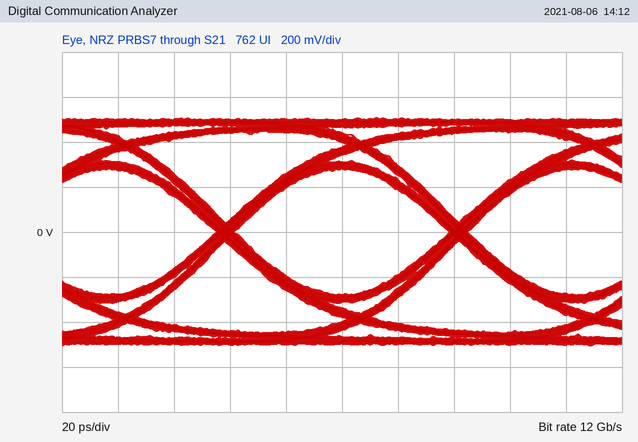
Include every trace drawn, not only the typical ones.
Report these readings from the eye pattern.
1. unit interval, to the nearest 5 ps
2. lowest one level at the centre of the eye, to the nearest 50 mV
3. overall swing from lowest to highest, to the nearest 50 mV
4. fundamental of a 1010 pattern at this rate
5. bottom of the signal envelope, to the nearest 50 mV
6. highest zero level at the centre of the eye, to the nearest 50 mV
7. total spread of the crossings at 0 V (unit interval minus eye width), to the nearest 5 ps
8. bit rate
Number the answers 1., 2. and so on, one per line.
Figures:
1. 85 ps
2. 300 mV
3. 1.00 V
4. 6 GHz
5. -500 mV
6. -300 mV
7. 5 ps
8. 12 Gb/s
